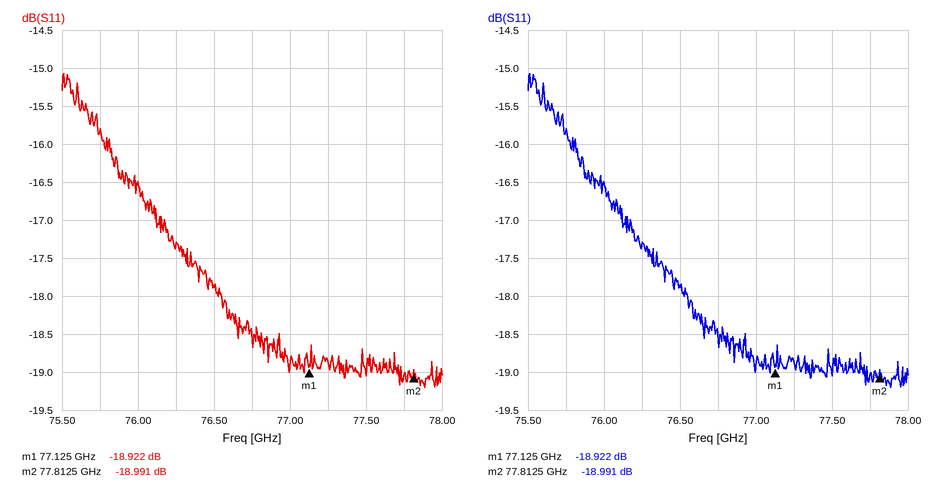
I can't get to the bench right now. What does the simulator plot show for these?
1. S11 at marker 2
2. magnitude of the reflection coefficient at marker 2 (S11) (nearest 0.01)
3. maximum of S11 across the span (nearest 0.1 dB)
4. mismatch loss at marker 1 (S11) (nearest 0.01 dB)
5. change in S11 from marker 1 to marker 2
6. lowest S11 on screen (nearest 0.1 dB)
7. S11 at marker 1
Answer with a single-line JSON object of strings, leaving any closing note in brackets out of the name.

{"S11 at marker 2": "-18.991 dB", "magnitude of the reflection coefficient at marker 2 (S11)": "0.11", "maximum of S11 across the span": "-15.1 dB", "mismatch loss at marker 1 (S11)": "0.06 dB", "change in S11 from marker 1 to marker 2": "-0.069 dB", "lowest S11 on screen": "-19.2 dB", "S11 at marker 1": "-18.922 dB"}
